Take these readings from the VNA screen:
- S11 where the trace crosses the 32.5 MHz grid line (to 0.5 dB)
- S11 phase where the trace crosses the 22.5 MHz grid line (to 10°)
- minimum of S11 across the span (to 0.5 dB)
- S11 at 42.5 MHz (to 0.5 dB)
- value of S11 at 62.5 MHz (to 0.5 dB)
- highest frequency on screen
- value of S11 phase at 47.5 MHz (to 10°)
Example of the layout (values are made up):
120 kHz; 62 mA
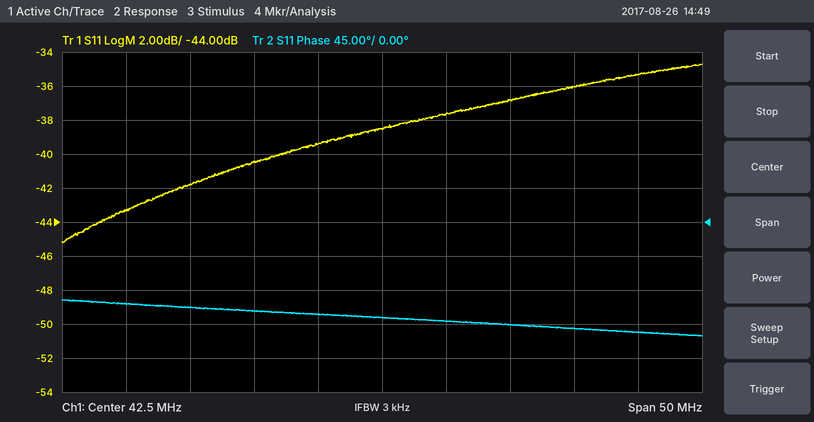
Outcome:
-40.5 dB; -110°; -45.0 dB; -38.5 dB; -35.5 dB; 67.5 MHz; -130°
